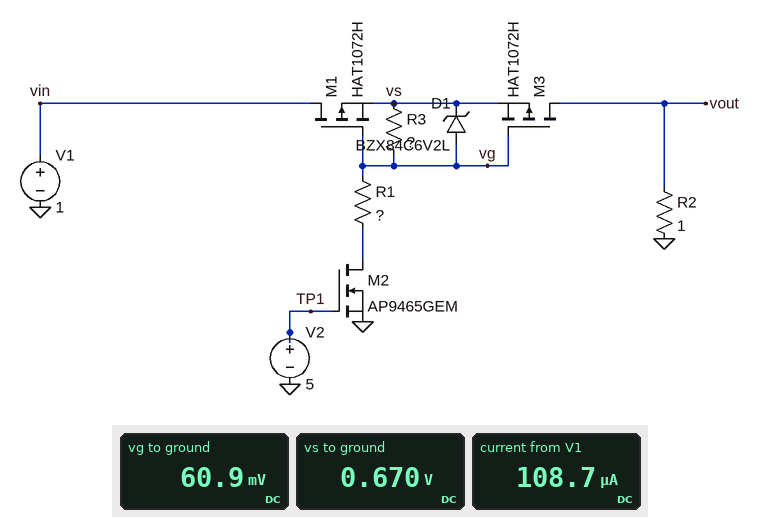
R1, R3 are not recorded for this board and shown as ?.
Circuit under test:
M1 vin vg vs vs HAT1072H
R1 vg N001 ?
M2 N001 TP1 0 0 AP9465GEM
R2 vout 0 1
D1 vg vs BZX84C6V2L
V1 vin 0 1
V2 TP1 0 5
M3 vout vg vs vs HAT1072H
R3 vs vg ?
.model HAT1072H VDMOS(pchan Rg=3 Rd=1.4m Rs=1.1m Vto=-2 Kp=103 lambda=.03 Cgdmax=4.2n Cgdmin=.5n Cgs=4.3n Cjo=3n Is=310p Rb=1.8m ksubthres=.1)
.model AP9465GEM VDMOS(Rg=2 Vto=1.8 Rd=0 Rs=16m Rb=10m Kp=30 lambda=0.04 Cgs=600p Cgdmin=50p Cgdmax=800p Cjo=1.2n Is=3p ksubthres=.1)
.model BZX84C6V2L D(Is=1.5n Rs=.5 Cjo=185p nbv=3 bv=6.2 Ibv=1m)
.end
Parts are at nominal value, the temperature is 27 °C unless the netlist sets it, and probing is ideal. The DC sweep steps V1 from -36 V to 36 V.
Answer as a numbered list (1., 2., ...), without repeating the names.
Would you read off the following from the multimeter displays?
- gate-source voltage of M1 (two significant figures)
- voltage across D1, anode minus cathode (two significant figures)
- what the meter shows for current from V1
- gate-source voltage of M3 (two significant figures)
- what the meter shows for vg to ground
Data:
1. -610 mV
2. -610 mV
3. 108.7 µA
4. -610 mV
5. 60.9 mV
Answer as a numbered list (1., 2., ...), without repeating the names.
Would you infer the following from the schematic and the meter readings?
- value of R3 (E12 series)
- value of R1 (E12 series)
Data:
1. 5.6 kΩ
2. 560 Ω
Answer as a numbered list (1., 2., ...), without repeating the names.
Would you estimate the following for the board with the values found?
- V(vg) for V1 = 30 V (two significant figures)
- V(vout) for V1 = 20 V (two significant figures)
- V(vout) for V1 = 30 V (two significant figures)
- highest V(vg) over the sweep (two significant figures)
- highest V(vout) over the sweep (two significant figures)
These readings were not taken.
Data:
1. 23 V
2. 20 V
3. 30 V
4. 29 V
5. 36 V
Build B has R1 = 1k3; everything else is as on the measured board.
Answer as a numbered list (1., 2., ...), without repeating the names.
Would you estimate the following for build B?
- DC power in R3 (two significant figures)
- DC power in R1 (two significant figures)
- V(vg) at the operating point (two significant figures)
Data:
1. 53 µW
2. 12 µW
3. 130 mV
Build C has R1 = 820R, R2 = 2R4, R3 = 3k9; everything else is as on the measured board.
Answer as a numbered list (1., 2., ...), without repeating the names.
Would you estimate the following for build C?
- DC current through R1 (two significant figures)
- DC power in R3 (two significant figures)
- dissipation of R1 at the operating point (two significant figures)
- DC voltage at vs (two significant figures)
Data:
1. 140 µA
2. 77 µW
3. 16 µW
4. 660 mV
